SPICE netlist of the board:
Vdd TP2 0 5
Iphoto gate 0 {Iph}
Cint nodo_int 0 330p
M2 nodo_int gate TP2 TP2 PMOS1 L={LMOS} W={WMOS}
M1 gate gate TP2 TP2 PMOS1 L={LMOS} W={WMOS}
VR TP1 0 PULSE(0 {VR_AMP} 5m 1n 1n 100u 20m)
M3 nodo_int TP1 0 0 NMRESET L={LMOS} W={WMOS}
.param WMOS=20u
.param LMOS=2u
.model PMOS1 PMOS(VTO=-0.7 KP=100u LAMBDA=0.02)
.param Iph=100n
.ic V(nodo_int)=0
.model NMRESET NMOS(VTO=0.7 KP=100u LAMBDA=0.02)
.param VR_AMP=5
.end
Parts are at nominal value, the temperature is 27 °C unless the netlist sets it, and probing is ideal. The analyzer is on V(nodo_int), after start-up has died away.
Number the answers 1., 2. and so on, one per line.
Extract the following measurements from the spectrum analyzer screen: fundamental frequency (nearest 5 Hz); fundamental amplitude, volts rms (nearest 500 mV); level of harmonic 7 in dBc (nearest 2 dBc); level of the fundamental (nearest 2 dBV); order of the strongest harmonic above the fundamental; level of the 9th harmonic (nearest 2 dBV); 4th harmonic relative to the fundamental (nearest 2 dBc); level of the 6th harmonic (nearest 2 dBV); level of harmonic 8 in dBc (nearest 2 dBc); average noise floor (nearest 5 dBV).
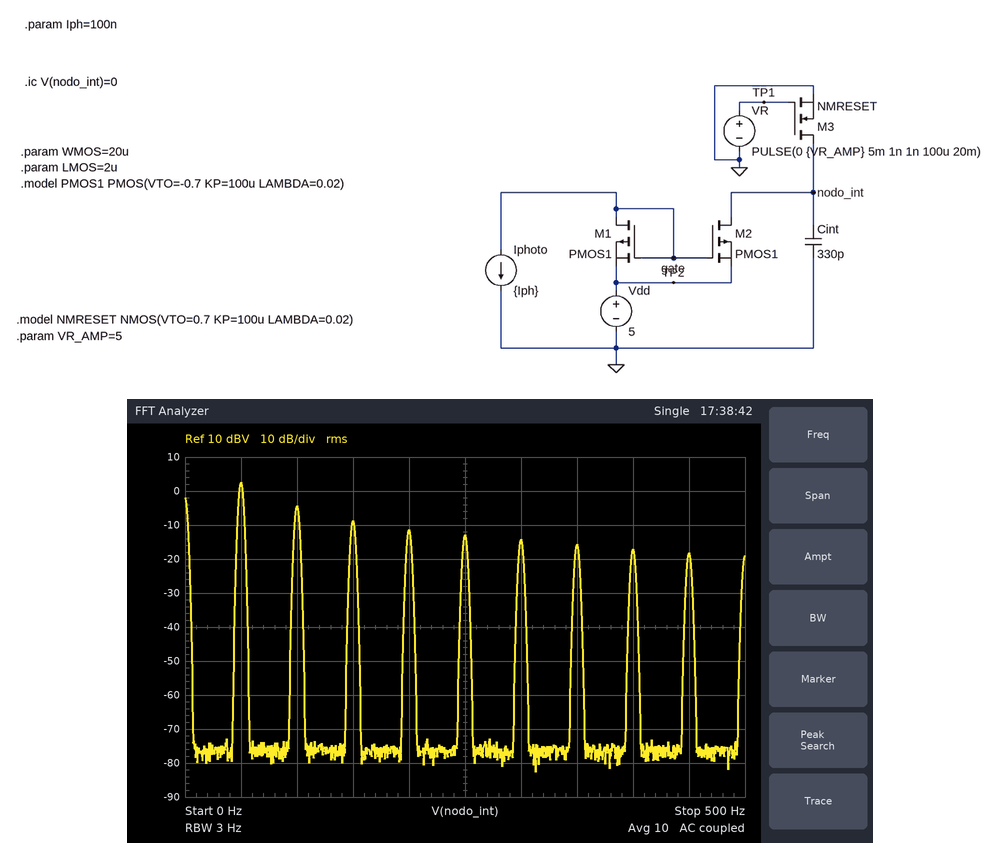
1. 50 Hz
2. 1.5 V
3. -18 dBc
4. 2 dBV
5. 2
6. -18 dBV
7. -14 dBc
8. -14 dBV
9. -20 dBc
10. -75 dBV
